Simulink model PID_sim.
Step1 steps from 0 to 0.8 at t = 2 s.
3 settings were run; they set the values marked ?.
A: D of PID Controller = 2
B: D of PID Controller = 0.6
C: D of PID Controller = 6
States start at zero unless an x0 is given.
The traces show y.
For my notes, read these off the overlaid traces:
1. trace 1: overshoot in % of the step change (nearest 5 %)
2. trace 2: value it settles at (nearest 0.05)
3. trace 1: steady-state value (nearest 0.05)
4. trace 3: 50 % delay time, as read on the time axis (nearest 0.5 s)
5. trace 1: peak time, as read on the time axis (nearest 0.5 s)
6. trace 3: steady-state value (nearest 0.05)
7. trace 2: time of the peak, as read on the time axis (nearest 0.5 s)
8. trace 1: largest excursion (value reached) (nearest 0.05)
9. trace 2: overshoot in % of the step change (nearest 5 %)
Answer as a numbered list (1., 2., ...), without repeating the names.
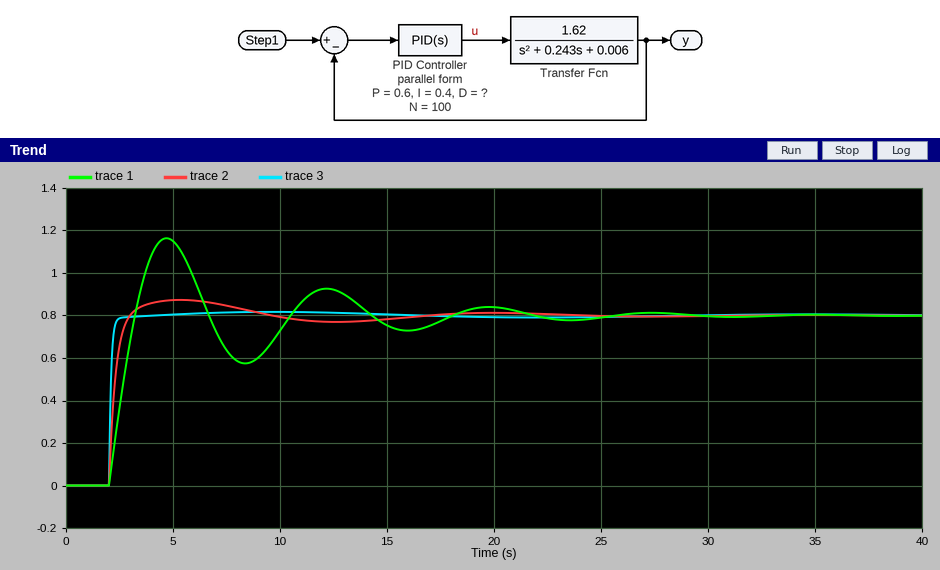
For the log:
1. 45 %
2. 0.80
3. 0.80
4. 2.0 s
5. 4.5 s
6. 0.80
7. 5.5 s
8. 1.15
9. 10 %
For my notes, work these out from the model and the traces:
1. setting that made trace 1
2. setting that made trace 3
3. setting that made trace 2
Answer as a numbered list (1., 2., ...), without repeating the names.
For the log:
1. B
2. C
3. A
